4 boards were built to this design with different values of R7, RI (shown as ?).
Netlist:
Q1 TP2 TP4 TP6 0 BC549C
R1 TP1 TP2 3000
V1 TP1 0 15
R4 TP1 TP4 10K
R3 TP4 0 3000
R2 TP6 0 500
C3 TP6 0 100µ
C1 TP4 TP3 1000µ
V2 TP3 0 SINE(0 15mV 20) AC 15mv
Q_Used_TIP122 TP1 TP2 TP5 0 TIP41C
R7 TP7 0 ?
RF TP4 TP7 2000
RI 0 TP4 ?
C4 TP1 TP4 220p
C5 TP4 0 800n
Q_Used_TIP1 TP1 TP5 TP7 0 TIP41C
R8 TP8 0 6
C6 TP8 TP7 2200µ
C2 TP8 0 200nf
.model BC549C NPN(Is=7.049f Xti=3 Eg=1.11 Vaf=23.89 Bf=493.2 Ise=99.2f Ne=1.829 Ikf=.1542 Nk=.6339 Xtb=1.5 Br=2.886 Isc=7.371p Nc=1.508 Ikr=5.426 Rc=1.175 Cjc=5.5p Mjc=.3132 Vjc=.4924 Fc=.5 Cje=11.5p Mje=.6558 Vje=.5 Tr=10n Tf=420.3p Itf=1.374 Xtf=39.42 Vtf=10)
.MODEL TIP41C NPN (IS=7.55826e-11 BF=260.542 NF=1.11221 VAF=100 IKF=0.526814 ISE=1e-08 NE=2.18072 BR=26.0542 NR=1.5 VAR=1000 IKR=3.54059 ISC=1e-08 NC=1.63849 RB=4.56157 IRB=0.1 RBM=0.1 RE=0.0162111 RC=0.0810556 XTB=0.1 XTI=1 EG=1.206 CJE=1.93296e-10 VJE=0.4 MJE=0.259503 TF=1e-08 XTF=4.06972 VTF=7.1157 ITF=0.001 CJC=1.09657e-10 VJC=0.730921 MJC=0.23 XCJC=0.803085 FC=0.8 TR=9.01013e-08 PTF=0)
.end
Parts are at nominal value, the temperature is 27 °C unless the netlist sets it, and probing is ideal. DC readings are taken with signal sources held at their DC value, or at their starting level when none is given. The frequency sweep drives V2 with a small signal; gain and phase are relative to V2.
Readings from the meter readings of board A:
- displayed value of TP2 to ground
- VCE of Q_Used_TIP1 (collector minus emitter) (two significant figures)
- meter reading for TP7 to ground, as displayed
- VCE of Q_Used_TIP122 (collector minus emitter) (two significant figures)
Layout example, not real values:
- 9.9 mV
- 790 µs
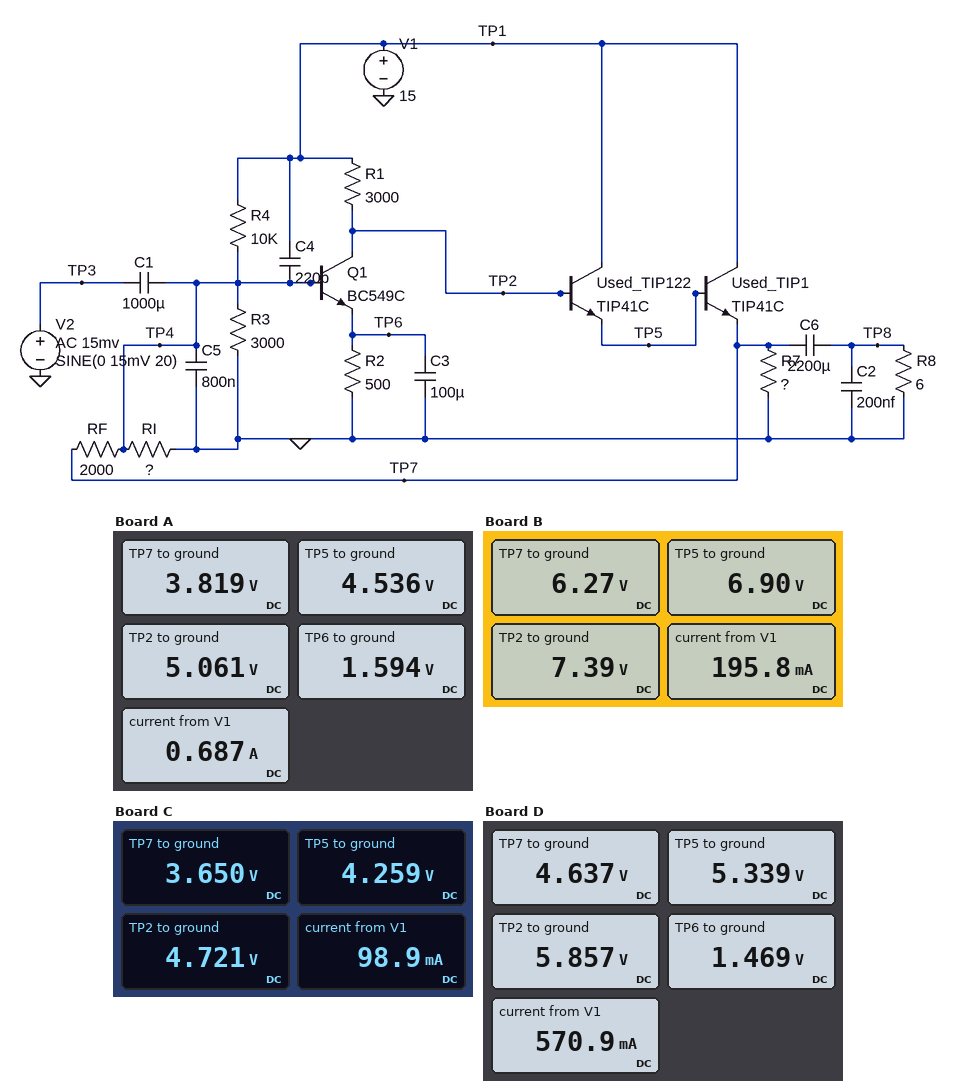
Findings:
- 5.061 V
- 11 V
- 3.819 V
- 10 V
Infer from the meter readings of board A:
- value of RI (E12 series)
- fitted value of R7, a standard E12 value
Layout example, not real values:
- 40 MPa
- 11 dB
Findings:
- 1.8 kΩ
- 5.6 Ω
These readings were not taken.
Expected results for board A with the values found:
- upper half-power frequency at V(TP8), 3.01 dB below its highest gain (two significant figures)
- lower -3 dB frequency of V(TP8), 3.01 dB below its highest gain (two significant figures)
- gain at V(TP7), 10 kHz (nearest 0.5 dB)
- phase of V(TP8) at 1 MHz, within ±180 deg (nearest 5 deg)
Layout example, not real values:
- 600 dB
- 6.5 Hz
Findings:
- 230 kHz
- 120 kHz
- 47.0 dB
- -45 deg
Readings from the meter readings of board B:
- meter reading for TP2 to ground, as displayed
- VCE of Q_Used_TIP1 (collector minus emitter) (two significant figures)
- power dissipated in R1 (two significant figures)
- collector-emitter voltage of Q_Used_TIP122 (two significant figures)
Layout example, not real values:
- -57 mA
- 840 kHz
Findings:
- 7.39 V
- 8.7 V
- 19 mW
- 8.1 V
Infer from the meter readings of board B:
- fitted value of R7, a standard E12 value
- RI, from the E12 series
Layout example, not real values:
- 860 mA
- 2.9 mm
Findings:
- 33 Ω
- 680 Ω
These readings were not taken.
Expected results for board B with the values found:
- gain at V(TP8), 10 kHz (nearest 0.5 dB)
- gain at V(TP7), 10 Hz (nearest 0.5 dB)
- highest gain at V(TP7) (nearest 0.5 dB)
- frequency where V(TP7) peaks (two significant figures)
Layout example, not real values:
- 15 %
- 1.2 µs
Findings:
- 46.0 dB
- 24.0 dB
- 54.0 dB
- 180 kHz
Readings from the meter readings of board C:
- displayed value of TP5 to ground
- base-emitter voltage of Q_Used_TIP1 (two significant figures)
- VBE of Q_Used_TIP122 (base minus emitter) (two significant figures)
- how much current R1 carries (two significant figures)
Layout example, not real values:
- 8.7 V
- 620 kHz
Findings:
- 4.259 V
- 610 mV
- 460 mV
- 3.4 mA
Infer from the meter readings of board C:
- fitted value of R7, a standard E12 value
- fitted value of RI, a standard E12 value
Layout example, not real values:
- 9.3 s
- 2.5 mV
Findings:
- 39 Ω
- 2.2 kΩ
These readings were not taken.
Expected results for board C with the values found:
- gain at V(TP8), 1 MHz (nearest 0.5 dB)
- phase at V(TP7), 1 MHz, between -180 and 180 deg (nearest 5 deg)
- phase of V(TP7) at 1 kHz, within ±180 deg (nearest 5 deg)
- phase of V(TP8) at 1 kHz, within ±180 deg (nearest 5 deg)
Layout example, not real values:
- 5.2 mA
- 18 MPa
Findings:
- 10.0 dB
- -45 deg
- -170 deg
- -170 deg
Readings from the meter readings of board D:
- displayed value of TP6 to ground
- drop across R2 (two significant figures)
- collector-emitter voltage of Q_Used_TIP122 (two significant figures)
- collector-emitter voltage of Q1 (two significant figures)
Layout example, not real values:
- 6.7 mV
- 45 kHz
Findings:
- 1.469 V
- 1.5 V
- 9.7 V
- 4.4 V
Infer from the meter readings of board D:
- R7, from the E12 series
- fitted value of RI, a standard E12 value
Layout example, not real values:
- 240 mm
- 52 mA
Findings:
- 8.2 Ω
- 1.2 kΩ
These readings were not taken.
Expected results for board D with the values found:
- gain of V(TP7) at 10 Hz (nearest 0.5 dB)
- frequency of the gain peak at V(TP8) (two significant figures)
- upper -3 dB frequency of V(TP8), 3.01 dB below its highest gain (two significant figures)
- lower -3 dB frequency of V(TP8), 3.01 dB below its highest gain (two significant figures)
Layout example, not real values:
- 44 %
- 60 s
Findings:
- 23.5 dB
- 190 kHz
- 220 kHz
- 140 kHz
